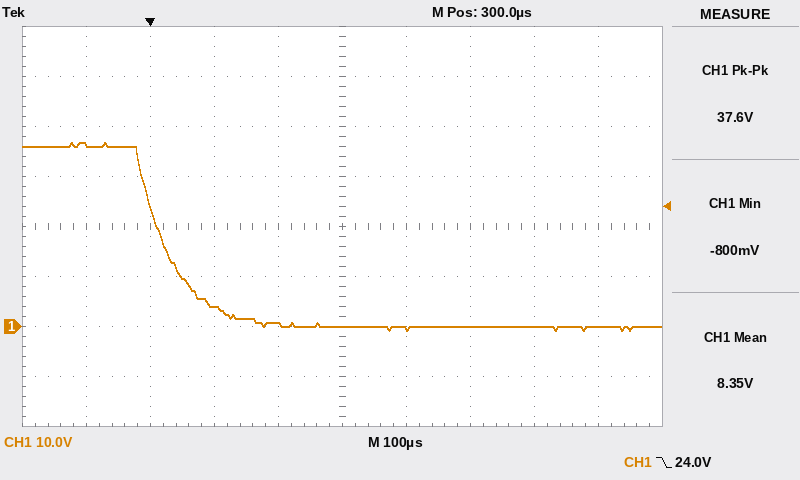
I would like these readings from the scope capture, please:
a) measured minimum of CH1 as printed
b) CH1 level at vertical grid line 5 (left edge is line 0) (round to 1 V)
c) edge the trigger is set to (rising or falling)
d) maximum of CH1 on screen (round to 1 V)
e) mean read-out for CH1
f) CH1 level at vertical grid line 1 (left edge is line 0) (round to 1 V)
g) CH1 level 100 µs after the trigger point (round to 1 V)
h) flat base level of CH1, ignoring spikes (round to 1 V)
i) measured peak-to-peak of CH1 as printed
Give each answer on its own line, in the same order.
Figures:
-800 mV
0 V
falling
37 V
8.35 V
36 V
4 V
0 V
37.6 V
